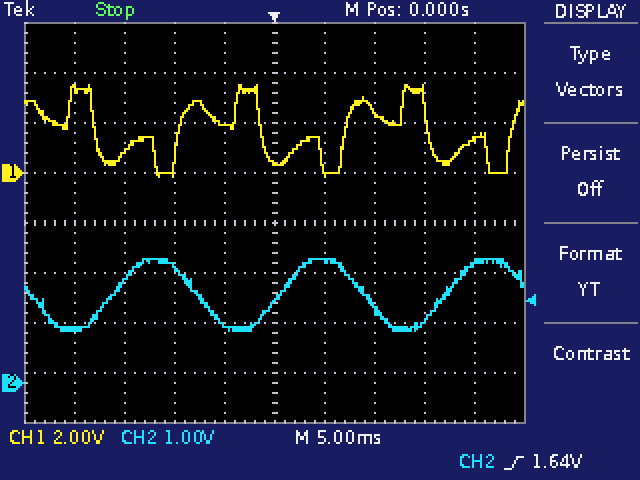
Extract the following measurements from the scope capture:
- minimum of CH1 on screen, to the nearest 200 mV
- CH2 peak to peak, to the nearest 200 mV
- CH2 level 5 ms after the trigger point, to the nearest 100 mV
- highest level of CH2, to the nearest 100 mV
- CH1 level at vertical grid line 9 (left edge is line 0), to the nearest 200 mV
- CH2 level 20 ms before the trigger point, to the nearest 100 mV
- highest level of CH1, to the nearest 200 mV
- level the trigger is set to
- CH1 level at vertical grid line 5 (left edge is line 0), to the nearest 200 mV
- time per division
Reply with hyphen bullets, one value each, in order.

- -200 mV
- 1.4 V
- 2.4 V
- 2.5 V
- 1.4 V
- 1.1 V
- 3.6 V
- 1.64 V
- 400 mV
- 5 ms
